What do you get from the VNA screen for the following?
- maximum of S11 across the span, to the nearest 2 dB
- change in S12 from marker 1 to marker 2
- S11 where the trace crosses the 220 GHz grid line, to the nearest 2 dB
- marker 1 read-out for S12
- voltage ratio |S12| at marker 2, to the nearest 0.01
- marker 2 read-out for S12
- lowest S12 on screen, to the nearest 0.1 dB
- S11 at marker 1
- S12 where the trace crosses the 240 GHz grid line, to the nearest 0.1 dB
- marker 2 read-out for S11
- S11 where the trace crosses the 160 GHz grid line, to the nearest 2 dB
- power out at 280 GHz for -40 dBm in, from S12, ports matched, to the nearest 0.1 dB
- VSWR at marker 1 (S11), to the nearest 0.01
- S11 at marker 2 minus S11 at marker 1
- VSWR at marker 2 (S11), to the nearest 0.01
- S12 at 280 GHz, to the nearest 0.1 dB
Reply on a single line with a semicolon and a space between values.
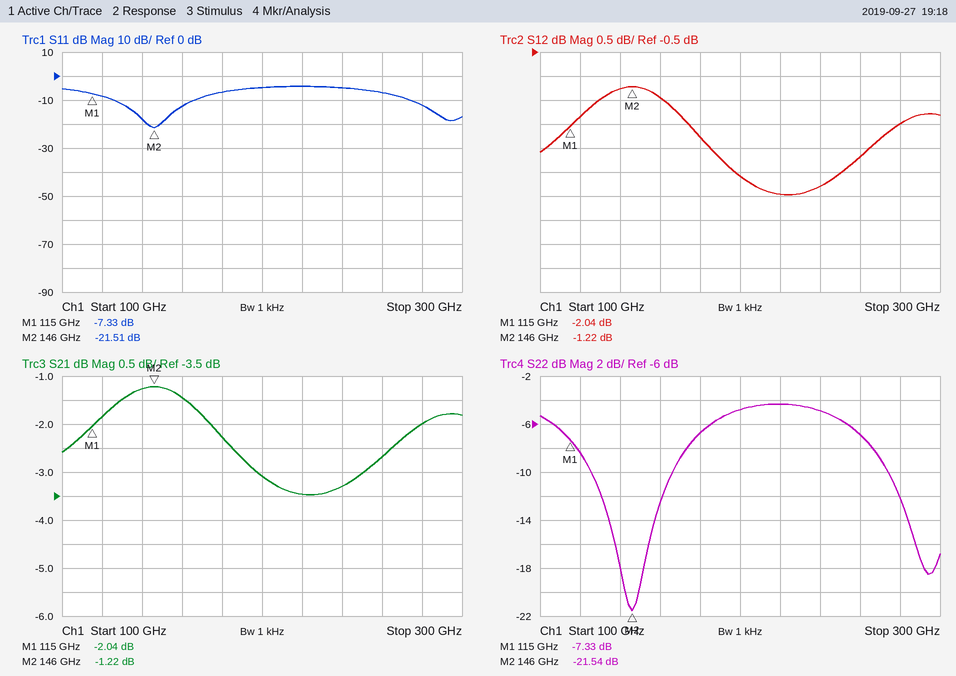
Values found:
-4 dB; 0.82 dB; -4 dB; -2.04 dB; 0.87; -1.22 dB; -3.5 dB; -7.33 dB; -3.3 dB; -21.51 dB; -12 dB; -42.0 dBm; 2.51; -14.18 dB; 1.18; -2.0 dB
